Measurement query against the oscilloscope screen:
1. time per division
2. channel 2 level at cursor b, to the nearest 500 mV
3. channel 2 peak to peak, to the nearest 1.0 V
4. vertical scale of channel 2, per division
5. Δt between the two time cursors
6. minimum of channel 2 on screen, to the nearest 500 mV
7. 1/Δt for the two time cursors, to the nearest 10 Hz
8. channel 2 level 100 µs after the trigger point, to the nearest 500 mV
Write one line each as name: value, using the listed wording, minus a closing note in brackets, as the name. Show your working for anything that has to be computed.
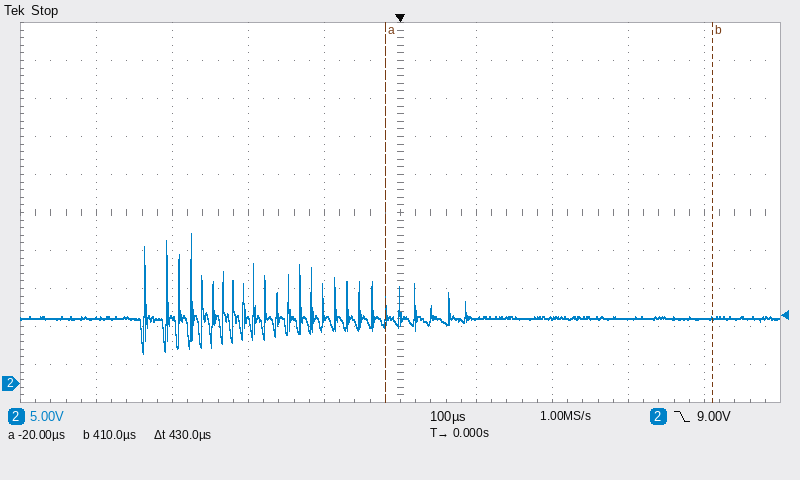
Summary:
time per division: 100 µs
channel 2 level at cursor b, to the nearest 500 mV: 8.5 V
channel 2 peak to peak, to the nearest 1.0 V: 16.0 V
vertical scale of channel 2, per division: 5 V
Δt between the two time cursors: 430 µs
minimum of channel 2 on screen, to the nearest 500 mV: 4.0 V
1/Δt for the two time cursors, to the nearest 10 Hz: 1 / 430 µs ≈ 2.33 kHz
channel 2 level 100 µs after the trigger point, to the nearest 500 mV: 8.5 V
